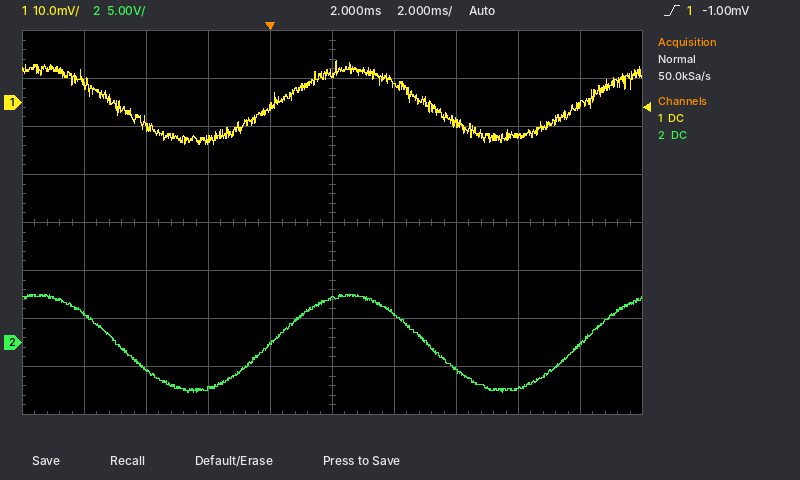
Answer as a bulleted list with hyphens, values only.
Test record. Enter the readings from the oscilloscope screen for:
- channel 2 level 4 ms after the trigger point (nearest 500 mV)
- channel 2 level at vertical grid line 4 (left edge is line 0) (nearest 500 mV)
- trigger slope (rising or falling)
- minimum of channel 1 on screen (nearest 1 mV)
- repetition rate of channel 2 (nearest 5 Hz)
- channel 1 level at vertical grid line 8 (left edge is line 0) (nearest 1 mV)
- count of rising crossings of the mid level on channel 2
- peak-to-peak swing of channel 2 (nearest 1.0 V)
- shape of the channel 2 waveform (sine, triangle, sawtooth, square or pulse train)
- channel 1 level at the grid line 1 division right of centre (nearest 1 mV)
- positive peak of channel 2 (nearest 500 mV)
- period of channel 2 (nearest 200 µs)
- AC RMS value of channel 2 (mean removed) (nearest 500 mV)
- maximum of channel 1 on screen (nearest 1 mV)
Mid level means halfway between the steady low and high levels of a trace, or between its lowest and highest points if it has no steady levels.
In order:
- 3.0 V
- 0.0 V
- rising
- -9 mV
- 100 Hz
- -7 mV
- 2
- 10.0 V
- sine
- 4 mV
- 5.0 V
- 10.0 ms
- 3.5 V
- 9 mV
